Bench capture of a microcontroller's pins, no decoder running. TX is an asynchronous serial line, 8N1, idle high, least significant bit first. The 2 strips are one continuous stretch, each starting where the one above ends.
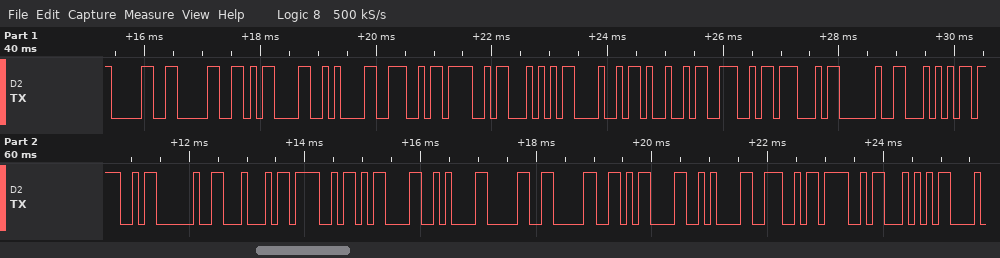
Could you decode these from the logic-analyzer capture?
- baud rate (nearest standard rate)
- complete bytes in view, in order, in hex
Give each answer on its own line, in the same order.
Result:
9600 baud
0x30 0x30 0x0D 0x0A 0x4E 0x4F 0x54 0x48 0x49 0x4E 0x47 0x20 0x54 0x4F 0x20 0x44 0x4F 0x0D 0x0A 0x30 0x30 0x0D 0x0A 0x4E 0x4F 0x54
